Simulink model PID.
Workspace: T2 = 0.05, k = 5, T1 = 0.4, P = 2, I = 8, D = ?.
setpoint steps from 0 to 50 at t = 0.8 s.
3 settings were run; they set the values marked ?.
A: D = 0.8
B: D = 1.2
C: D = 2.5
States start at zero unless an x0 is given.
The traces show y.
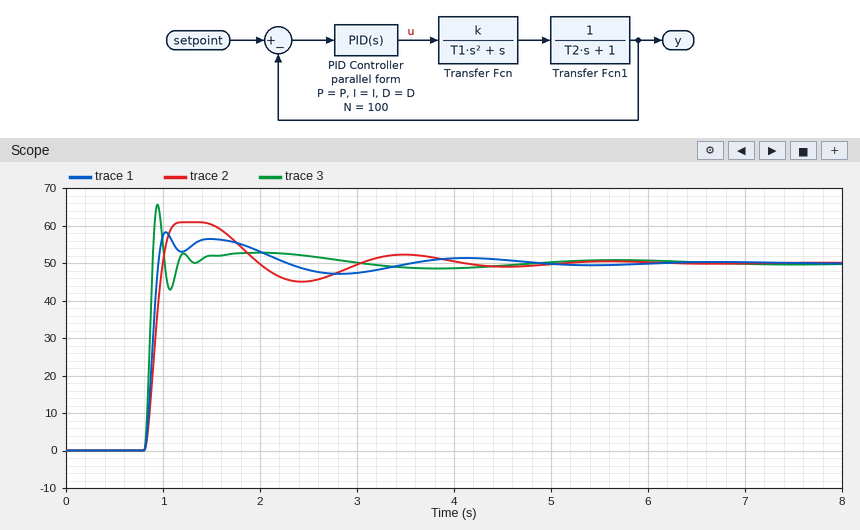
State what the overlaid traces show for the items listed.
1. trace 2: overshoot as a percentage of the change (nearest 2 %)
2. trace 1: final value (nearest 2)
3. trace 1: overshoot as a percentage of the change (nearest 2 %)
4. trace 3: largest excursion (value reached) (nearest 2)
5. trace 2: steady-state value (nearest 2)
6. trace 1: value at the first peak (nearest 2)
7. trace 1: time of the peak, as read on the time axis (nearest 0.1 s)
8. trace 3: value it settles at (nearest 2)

22 %
50
16 %
66
50
58
1.0 s
50
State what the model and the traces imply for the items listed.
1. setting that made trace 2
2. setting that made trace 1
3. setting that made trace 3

A
B
C
